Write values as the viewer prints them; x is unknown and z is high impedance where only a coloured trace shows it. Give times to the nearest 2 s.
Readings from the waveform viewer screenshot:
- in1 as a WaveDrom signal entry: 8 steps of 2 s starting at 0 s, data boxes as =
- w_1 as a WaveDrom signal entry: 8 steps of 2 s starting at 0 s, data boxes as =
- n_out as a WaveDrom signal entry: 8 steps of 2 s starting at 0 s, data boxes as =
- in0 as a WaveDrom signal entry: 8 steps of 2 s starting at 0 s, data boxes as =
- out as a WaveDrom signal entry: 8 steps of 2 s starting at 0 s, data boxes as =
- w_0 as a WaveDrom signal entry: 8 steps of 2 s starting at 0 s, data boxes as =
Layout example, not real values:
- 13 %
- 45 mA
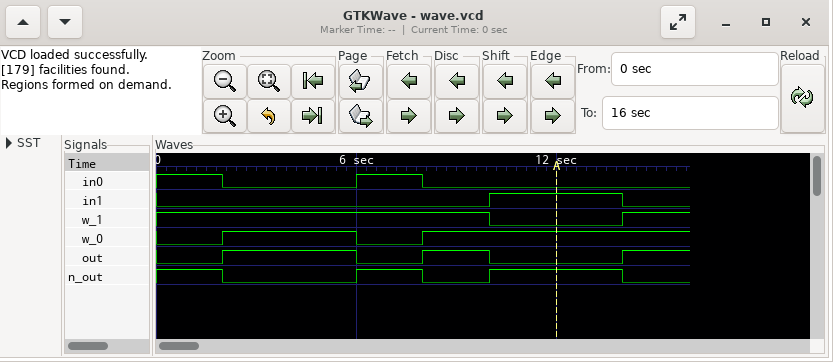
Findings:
- {name: 'in1', wave: '0....1.0'}
- {name: 'w_1', wave: '1....0.1'}
- {name: 'n_out', wave: '10.101.0'}
- {name: 'in0', wave: '10.10...'}
- {name: 'out', wave: '01.010.1'}
- {name: 'w_0', wave: '01.01...'}
